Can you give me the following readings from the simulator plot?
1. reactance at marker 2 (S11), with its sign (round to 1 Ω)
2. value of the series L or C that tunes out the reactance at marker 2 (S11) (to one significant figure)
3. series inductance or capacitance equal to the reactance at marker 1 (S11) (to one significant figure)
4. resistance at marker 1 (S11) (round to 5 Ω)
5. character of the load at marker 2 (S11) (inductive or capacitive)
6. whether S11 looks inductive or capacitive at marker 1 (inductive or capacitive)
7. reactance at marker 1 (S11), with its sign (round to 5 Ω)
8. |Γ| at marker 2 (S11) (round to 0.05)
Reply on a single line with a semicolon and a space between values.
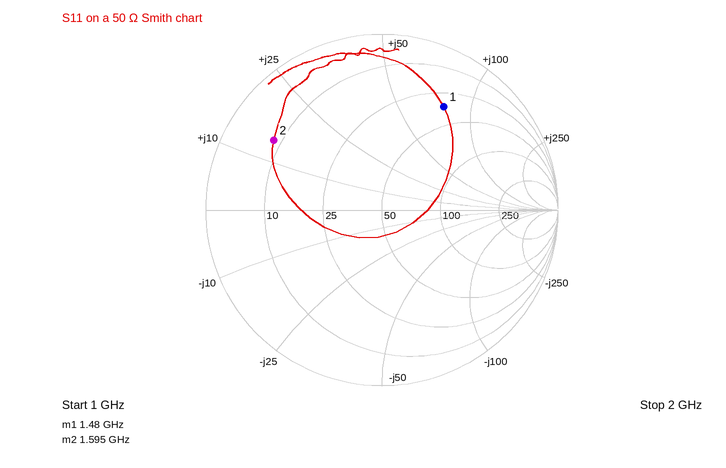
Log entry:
+14 Ω; 7 pF; 8 nH; 35 Ω; inductive; inductive; +75 Ω; 0.75
